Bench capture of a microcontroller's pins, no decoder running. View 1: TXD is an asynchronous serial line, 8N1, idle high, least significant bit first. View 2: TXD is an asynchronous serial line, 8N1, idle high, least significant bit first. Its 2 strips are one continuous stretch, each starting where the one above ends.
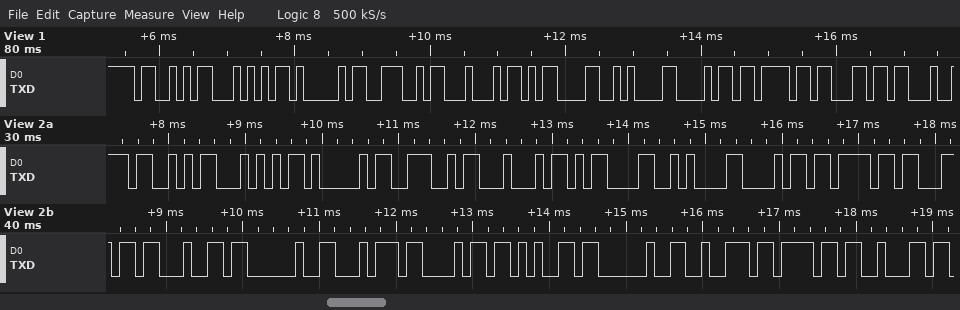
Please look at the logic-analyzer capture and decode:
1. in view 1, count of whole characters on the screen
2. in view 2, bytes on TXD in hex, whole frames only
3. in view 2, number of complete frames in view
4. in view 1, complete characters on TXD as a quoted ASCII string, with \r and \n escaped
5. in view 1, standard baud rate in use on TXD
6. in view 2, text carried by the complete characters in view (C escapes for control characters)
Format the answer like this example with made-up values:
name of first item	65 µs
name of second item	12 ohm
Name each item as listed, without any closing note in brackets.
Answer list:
in view 1, count of whole characters on the screen	10
in view 2, bytes on TXD in hex, whole frames only	53 54 41 4E 44 0D 0A 68 6F 6C 64 20 74 68 65 20 72 6F 62
in view 2, number of complete frames in view	19
in view 1, complete characters on TXD as a quoted ASCII string, with \r and \n escaped	"STAND\r\nhol"
in view 1, standard baud rate in use on TXD	9600 baud
in view 2, text carried by the complete characters in view	"STAND\r\nhold the rob"
